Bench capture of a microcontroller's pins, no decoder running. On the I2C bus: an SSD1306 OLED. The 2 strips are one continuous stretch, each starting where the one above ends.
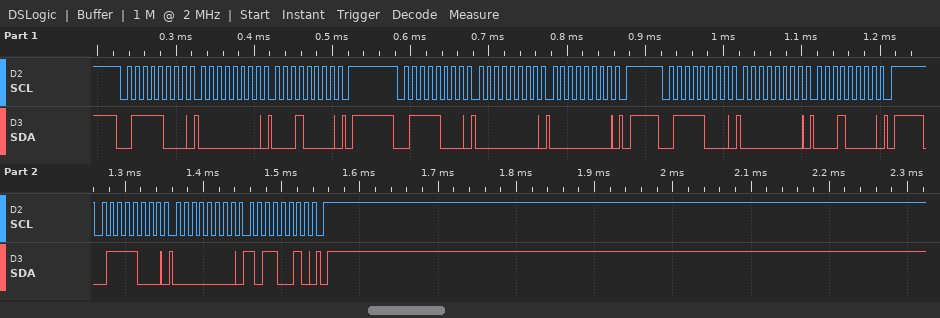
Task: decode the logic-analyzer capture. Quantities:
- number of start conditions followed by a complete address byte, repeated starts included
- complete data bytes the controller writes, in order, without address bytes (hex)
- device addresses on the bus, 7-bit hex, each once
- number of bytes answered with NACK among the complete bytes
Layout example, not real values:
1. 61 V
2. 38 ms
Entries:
1. 4
2. 00 10 00 00 00 10 00 B2
3. 0x3C
4. 0
